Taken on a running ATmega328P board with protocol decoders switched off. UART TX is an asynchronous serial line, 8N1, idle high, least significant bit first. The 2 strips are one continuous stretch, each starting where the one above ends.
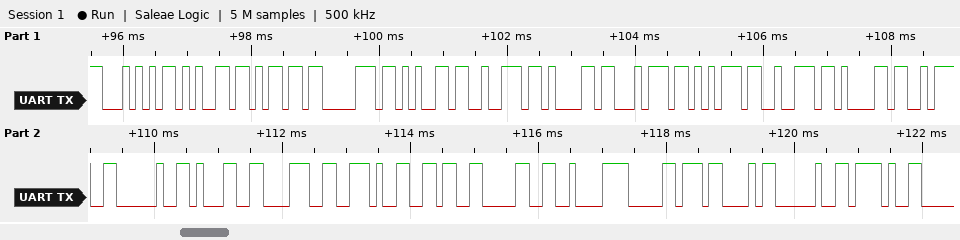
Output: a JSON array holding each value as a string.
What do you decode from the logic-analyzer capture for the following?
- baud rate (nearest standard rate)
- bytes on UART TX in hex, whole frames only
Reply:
["9600 baud", "54 65 6D 70 65 72 61 74 75 72 61 3A 20 31 38 2E 36 30 C2 B0 43 20 2F"]
